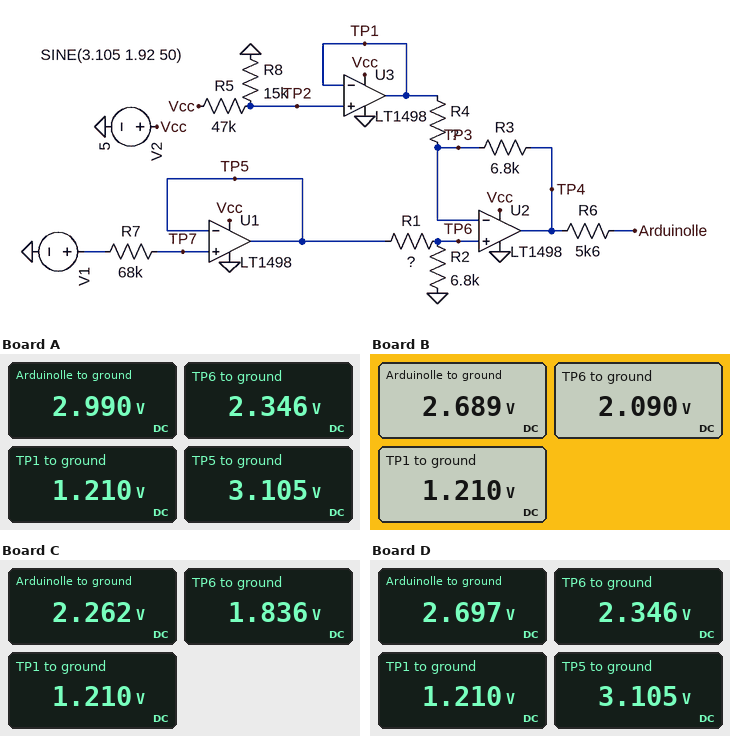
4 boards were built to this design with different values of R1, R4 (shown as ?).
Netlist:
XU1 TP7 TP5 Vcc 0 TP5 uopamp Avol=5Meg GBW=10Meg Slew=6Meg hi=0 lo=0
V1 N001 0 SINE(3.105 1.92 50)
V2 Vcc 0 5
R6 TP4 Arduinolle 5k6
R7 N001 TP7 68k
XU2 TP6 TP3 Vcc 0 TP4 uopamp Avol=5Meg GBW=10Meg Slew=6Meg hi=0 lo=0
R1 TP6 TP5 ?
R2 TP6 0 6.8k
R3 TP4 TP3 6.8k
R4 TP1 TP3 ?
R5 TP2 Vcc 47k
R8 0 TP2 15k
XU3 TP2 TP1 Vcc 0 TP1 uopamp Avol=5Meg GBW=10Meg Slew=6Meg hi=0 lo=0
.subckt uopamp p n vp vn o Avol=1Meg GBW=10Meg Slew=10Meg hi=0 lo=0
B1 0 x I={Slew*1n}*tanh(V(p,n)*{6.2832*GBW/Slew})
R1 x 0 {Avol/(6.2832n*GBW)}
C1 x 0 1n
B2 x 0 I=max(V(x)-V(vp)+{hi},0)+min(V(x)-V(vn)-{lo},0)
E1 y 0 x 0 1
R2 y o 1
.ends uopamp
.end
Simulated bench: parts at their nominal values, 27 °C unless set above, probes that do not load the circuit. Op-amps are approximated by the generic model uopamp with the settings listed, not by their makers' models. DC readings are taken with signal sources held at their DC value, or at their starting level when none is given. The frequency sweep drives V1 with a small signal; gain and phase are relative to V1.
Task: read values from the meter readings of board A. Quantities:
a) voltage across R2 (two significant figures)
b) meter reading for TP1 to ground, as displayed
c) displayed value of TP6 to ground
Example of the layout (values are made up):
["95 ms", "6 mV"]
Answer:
["2.3 V", "1.210 V", "2.346 V"]
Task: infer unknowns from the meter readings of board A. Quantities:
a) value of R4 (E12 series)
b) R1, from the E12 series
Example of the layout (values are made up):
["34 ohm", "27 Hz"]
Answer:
["12 kΩ", "2.2 kΩ"]
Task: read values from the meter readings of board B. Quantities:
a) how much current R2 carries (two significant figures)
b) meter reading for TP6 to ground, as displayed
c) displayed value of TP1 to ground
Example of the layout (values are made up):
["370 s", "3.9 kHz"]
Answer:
["310 µA", "2.090 V", "1.210 V"]
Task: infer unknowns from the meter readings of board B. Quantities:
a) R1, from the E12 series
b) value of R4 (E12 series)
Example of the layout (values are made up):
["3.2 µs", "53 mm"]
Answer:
["3.3 kΩ", "10 kΩ"]
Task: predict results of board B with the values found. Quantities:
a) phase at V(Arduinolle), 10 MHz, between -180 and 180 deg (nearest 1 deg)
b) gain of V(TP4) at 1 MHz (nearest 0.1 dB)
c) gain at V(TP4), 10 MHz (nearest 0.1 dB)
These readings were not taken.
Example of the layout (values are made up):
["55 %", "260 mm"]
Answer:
["-104 deg", "0.9 dB", "-7.8 dB"]
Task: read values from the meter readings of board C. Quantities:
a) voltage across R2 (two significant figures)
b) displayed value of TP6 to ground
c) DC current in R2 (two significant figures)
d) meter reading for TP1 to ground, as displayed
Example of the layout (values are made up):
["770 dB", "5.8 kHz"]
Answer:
["1.8 V", "1.836 V", "270 µA", "1.210 V"]
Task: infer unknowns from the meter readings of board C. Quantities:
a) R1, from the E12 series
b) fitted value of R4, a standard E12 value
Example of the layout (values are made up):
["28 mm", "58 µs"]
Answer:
["4.7 kΩ", "10 kΩ"]
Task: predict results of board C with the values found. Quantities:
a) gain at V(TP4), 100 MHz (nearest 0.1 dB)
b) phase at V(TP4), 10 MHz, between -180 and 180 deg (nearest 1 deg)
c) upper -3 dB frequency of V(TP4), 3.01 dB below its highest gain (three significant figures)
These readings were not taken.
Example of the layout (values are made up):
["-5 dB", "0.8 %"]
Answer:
["-44.6 dB", "-104 deg", "4.74 MHz"]
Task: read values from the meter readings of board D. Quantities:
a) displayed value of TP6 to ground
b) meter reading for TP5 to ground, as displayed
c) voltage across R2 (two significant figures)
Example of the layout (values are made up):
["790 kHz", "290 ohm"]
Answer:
["2.346 V", "3.105 V", "2.3 V"]
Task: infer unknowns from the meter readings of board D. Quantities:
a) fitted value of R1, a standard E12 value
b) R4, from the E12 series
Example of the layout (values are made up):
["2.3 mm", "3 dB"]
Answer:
["2.2 kΩ", "22 kΩ"]
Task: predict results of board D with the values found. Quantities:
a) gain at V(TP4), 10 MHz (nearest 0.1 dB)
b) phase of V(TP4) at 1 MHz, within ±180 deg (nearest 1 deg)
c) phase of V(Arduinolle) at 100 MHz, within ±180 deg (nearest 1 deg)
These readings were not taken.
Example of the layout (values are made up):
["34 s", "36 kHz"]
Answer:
["-7.4 dB", "-13 deg", "-170 deg"]
